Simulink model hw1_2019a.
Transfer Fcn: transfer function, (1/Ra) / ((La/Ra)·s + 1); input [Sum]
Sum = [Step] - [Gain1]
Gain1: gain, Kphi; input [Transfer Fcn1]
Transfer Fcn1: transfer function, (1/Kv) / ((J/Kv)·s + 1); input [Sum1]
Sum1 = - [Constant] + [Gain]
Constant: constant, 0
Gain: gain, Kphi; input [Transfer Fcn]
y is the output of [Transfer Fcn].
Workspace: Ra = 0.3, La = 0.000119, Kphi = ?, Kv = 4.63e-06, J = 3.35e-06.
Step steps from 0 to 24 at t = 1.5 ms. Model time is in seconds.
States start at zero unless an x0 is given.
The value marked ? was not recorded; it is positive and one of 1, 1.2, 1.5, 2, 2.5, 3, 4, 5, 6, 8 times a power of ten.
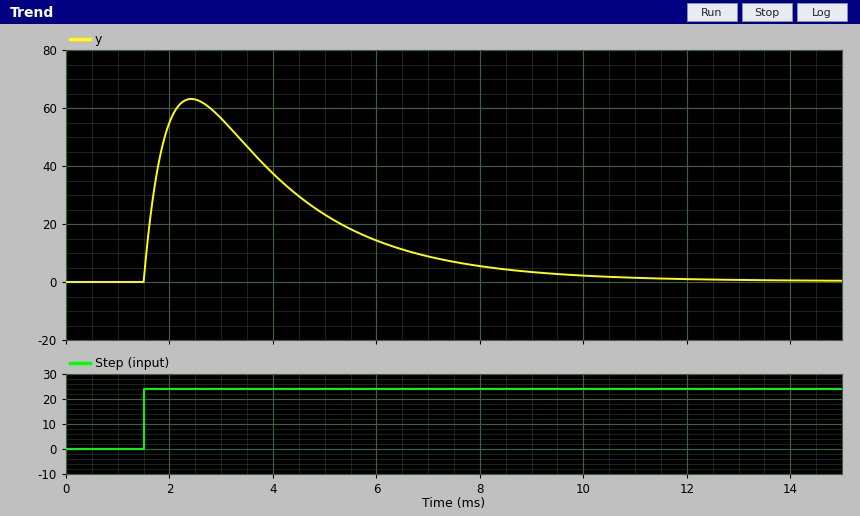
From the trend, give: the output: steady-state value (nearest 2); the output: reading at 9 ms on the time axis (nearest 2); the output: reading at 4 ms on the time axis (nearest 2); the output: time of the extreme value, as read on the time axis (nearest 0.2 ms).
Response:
0
4
38
2.4 ms
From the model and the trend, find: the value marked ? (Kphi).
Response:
0.02
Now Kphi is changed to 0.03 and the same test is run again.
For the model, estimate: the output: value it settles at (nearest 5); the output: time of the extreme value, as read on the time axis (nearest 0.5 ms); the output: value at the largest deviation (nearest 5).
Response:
0
2.0 ms
55
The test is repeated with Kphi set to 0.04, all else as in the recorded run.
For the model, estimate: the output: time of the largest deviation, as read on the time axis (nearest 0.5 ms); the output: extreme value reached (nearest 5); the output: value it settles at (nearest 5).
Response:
2.0 ms
50
0
